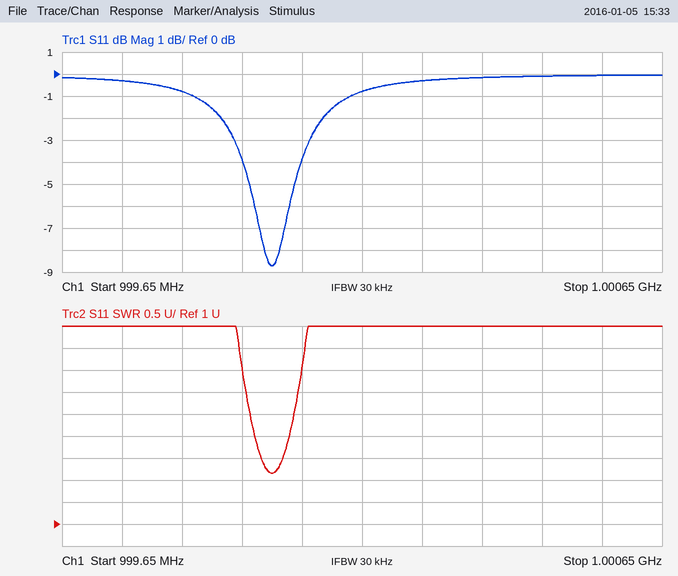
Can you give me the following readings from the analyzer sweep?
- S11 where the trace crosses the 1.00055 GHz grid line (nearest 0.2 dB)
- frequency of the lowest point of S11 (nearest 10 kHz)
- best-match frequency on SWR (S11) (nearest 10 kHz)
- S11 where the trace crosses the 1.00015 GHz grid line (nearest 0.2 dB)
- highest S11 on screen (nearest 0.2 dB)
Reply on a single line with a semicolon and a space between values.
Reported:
0.0 dB; 1.00000 GHz; 1.00000 GHz; -0.8 dB; 0.0 dB
